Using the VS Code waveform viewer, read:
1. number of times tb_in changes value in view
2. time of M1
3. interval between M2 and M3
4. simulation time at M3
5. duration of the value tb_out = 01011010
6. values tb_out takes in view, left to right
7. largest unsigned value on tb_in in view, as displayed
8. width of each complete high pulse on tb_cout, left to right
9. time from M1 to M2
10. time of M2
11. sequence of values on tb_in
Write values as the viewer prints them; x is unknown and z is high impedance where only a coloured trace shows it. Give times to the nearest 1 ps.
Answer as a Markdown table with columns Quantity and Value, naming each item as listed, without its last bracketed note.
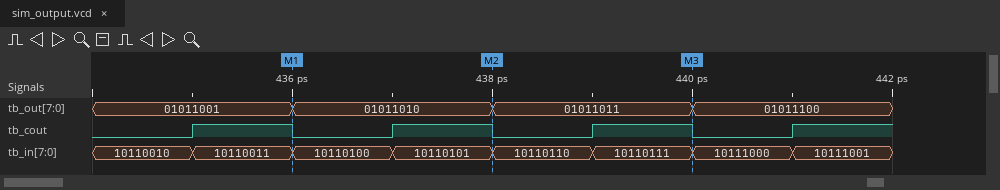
| Quantity | Value |
|---|---|
| number of times tb_in changes value in view | 7 |
| time of M1 | 436 ps |
| interval between M2 and M3 | 2 ps |
| simulation time at M3 | 440 ps |
| duration of the value tb_out = 01011010 | 2 ps |
| values tb_out takes in view, left to right | 01011001, 01011010, 01011011, 01011100 |
| largest unsigned value on tb_in in view, as displayed | 10111001 |
| width of each complete high pulse on tb_cout, left to right | 1 ps, 1 ps, 1 ps |
| time from M1 to M2 | 2 ps |
| time of M2 | 438 ps |
| sequence of values on tb_in | 10110010, 10110011, 10110100, 10110101, 10110110, 10110111, 10111000, 10111001 |
